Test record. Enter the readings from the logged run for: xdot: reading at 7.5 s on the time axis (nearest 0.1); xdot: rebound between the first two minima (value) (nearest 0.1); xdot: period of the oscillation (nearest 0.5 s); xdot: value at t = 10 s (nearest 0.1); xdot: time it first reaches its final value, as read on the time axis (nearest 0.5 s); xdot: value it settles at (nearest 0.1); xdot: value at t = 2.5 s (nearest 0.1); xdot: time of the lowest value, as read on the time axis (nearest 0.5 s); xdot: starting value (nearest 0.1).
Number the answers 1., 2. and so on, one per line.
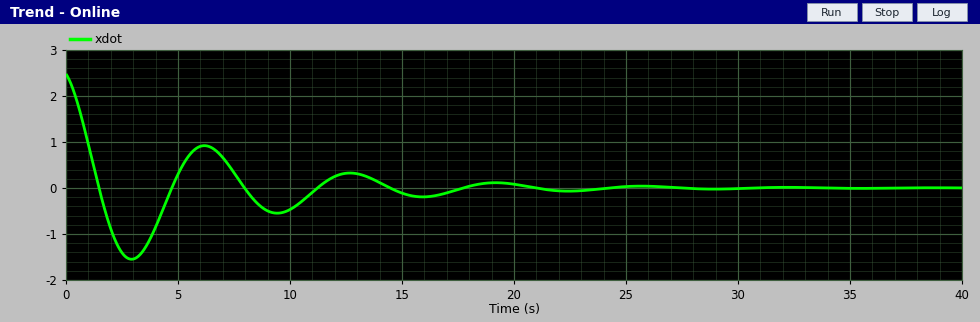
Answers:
1. 0.3
2. 0.9
3. 6.5 s
4. -0.5
5. 1.5 s
6. 0.0
7. -1.4
8. 3.0 s
9. 2.5
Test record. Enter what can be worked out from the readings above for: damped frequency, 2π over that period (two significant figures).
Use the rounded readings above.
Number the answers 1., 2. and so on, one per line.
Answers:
1. 0.97 rad/s
